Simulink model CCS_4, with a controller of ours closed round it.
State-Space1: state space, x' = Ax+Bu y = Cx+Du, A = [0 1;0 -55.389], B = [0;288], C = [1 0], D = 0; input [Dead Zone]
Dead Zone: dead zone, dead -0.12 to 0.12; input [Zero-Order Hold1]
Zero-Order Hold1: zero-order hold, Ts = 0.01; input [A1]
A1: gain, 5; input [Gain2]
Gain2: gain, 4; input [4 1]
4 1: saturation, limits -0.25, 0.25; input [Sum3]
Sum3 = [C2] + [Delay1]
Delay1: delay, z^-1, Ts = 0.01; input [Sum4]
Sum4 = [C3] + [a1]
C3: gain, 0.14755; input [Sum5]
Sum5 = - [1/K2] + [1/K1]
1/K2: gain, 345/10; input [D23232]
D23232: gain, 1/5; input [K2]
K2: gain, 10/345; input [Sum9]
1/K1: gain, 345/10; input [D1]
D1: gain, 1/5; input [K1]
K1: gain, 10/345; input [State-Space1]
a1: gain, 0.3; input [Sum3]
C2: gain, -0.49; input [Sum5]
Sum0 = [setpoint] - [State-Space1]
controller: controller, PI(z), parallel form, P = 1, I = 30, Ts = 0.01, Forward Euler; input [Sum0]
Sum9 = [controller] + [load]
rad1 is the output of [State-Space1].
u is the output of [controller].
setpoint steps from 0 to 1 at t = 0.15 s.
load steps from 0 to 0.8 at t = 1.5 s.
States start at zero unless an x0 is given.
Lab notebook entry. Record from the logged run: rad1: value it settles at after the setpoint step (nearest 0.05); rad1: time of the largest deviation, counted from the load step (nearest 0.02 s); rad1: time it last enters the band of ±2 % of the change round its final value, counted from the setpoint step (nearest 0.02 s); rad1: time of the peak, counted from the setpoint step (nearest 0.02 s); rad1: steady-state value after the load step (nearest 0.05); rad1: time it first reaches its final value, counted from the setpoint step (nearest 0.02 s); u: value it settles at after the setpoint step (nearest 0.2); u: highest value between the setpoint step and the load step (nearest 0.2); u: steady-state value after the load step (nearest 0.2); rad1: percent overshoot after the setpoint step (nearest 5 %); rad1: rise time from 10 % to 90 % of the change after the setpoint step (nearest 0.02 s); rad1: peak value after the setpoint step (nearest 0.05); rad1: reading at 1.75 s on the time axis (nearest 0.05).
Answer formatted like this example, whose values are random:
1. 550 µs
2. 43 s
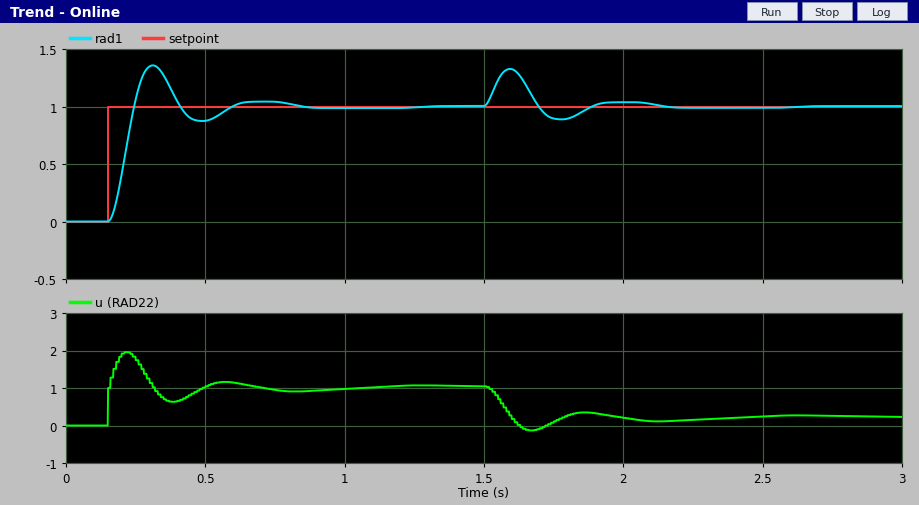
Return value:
1. 1.00
2. 0.10 s
3. 0.66 s
4. 0.16 s
5. 1.00
6. 0.10 s
7. 1.0
8. 2.0
9. 0.2
10. 35 %
11. 0.06 s
12. 1.35
13. 0.90
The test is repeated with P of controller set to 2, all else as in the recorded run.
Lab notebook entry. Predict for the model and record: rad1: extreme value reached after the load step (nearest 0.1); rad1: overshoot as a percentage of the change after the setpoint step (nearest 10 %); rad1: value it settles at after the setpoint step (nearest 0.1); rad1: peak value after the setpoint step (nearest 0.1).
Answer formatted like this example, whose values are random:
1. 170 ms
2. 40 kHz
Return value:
1. 1.3
2. 20 %
3. 1.0
4. 1.2
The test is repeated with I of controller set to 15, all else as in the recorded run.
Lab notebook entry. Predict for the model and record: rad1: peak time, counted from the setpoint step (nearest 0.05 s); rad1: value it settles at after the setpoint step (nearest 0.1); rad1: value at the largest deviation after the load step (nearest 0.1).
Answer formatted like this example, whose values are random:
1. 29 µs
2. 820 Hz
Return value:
1. 0.35 s
2. 1.0
3. 1.3
